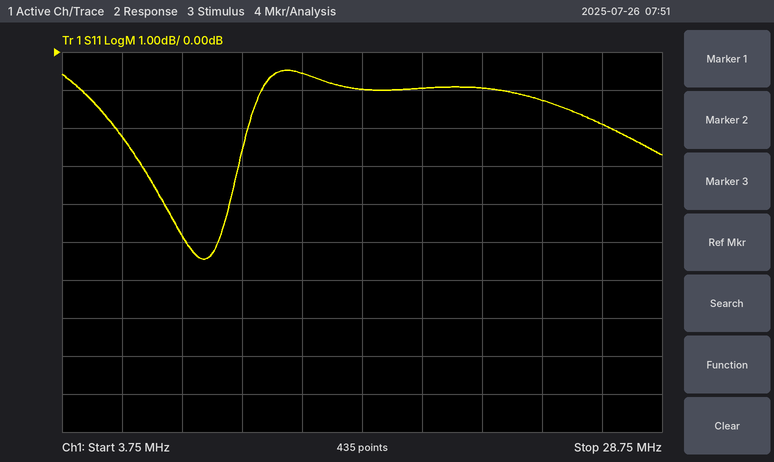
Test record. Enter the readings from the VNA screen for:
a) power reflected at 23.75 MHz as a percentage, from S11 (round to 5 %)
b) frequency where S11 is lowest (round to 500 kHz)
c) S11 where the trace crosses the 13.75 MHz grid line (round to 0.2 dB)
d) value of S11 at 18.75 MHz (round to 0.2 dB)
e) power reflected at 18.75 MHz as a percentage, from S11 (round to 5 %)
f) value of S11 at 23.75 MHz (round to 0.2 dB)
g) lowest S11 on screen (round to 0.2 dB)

75 %
9.5 MHz
-0.6 dB
-1.0 dB
80 %
-1.2 dB
-5.4 dB
